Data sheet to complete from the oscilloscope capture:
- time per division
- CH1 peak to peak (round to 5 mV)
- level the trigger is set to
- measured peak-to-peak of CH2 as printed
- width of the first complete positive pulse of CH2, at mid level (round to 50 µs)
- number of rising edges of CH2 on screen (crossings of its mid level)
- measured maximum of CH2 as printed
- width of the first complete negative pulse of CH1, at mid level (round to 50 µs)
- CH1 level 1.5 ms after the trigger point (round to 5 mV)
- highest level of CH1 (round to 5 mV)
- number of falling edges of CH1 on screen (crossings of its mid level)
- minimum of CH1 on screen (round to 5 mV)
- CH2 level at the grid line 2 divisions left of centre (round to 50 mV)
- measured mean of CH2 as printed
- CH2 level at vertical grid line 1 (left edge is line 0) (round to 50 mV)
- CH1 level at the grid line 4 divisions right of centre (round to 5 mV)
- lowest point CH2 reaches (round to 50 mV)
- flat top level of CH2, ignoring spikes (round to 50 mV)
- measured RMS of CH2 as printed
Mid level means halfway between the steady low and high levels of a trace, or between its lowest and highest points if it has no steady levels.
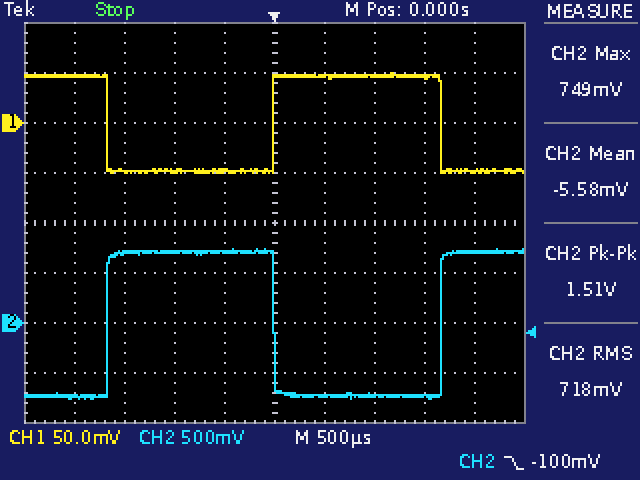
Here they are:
500 µs
100 mV
-100 mV
1.51 V
1.65 ms
2
749 mV
1.65 ms
45 mV
50 mV
2
-50 mV
700 mV
-5.58 mV
-750 mV
-50 mV
-750 mV
700 mV
718 mV
